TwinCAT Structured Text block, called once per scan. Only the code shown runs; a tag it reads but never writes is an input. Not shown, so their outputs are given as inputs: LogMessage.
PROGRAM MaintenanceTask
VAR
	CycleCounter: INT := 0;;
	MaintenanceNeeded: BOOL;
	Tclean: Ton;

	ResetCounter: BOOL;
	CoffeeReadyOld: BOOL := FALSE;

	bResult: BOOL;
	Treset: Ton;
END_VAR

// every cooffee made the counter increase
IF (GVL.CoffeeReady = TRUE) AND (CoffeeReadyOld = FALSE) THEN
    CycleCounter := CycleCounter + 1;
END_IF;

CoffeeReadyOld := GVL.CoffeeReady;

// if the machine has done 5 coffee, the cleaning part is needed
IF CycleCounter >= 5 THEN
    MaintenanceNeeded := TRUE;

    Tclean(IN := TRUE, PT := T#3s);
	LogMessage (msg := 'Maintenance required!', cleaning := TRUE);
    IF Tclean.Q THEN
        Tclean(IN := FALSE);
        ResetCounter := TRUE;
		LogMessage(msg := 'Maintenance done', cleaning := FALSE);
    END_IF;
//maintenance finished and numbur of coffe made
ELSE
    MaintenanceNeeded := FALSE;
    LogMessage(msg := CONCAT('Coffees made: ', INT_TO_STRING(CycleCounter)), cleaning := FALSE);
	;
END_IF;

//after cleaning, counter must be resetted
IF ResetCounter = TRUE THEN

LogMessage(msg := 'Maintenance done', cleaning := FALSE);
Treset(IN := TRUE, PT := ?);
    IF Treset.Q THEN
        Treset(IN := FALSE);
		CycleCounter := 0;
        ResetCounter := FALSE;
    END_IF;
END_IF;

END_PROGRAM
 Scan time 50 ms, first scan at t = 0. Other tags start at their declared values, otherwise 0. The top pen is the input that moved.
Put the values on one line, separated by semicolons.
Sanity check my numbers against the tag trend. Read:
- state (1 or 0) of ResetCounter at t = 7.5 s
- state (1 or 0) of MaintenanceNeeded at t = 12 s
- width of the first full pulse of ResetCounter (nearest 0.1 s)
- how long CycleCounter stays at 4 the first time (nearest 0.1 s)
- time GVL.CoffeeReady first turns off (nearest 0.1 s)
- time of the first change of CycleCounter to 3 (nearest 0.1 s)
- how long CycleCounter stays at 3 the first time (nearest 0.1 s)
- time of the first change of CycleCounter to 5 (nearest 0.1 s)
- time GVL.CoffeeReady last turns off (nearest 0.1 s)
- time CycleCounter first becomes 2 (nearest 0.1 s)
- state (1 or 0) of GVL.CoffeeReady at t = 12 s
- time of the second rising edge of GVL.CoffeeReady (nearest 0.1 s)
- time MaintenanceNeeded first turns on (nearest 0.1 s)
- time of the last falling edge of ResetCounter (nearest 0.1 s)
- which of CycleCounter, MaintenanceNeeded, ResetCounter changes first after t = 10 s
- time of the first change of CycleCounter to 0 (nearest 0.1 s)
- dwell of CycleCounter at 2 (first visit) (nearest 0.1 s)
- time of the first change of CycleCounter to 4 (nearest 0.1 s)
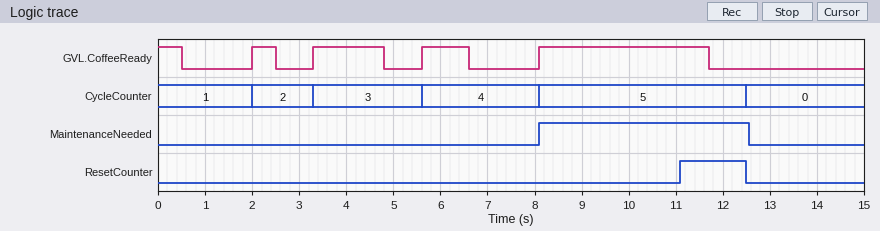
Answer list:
0; 1; 1.4 s; 2.5 s; 0.5 s; 3.3 s; 2.3 s; 8.1 s; 11.7 s; 2.0 s; 0; 3.3 s; 8.1 s; 12.5 s; ResetCounter; 12.5 s; 1.3 s; 5.6 s
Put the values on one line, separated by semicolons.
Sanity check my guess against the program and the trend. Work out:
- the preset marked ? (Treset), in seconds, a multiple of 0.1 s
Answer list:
1.4 s
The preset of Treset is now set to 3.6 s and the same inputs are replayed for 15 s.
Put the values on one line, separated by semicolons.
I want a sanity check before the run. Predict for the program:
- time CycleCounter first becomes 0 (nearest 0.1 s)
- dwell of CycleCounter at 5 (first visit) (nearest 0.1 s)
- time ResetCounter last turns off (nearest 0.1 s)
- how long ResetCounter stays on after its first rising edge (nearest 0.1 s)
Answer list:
14.7 s; 6.6 s; 14.7 s; 3.6 s
